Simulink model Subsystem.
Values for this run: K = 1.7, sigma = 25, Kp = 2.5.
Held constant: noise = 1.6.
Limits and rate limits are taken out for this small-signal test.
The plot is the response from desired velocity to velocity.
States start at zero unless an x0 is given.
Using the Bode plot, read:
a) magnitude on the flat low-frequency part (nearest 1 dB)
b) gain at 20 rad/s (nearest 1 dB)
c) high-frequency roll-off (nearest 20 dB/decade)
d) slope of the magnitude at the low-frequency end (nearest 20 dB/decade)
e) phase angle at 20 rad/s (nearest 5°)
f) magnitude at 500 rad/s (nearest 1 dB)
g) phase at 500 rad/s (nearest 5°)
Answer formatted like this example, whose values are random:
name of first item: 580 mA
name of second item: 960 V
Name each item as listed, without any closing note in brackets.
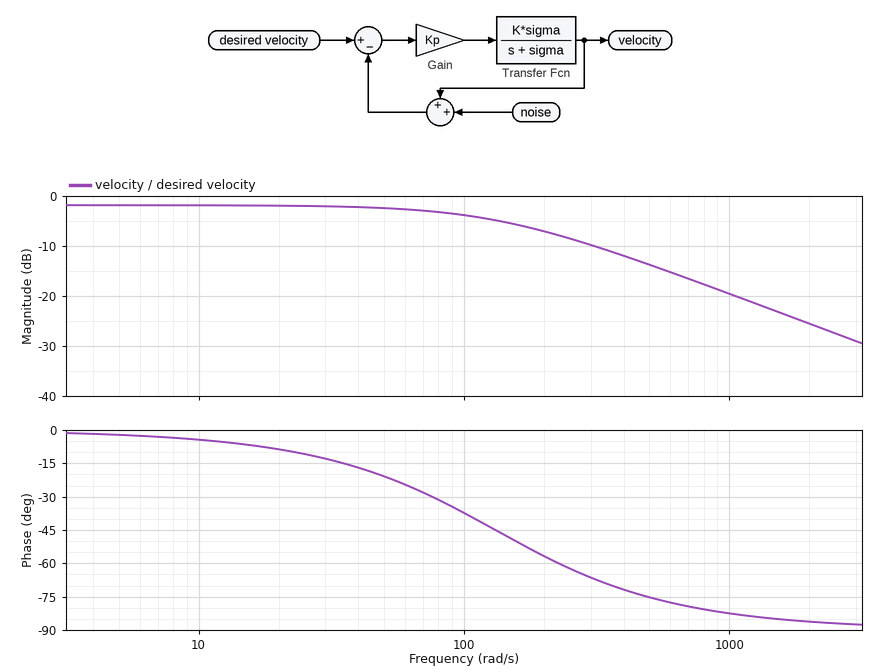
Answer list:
magnitude on the flat low-frequency part: -2 dB
gain at 20 rad/s: -2 dB
high-frequency roll-off: -20 dB/decade
slope of the magnitude at the low-frequency end: 0 dB/decade
phase angle at 20 rad/s: -10°
magnitude at 500 rad/s: -14 dB
phase at 500 rad/s: -75°
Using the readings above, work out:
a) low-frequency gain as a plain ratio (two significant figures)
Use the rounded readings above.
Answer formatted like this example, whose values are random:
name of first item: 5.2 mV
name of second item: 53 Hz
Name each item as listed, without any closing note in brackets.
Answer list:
low-frequency gain as a plain ratio: 0.79
